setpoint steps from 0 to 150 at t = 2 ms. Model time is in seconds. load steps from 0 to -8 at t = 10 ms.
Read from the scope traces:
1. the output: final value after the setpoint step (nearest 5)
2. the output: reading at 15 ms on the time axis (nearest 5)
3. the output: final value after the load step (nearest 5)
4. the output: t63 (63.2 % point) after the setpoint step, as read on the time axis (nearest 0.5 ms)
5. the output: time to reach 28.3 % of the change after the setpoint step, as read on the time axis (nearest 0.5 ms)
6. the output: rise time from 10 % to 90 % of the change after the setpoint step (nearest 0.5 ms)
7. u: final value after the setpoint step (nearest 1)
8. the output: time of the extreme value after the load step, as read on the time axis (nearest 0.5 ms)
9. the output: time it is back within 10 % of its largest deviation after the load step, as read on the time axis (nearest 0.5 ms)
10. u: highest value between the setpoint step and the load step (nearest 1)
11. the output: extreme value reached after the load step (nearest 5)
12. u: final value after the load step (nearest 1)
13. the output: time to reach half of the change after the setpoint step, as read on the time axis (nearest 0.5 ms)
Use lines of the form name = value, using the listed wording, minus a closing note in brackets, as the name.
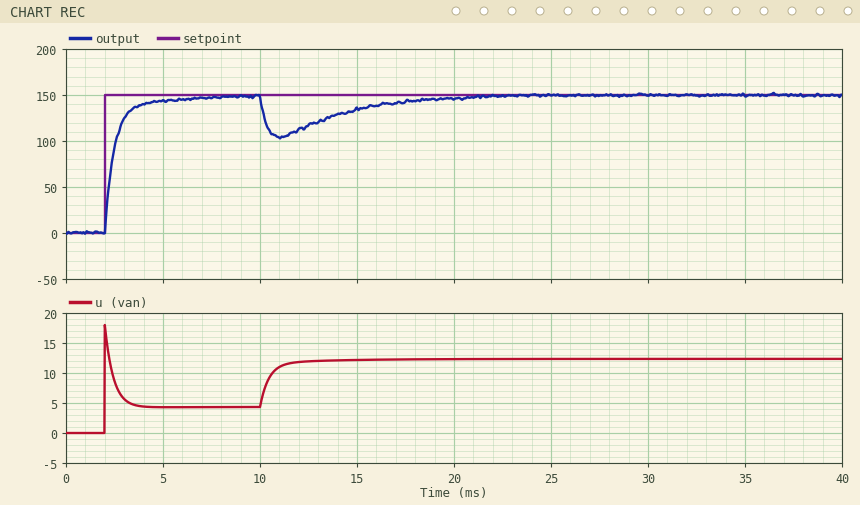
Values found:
the output: final value after the setpoint step = 150
the output: reading at 15 ms on the time axis = 135
the output: final value after the load step = 150
the output: t63 (63.2 % point) after the setpoint step, as read on the time axis = 2.5 ms
the output: time to reach 28.3 % of the change after the setpoint step, as read on the time axis = 2.0 ms
the output: rise time from 10 % to 90 % of the change after the setpoint step = 1.5 ms
u: final value after the setpoint step = 4
the output: time of the extreme value after the load step, as read on the time axis = 11.0 ms
the output: time it is back within 10 % of its largest deviation after the load step, as read on the time axis = 19.0 ms
u: highest value between the setpoint step and the load step = 18
the output: extreme value reached after the load step = 105
u: final value after the load step = 12
the output: time to reach half of the change after the setpoint step, as read on the time axis = 2.5 ms
